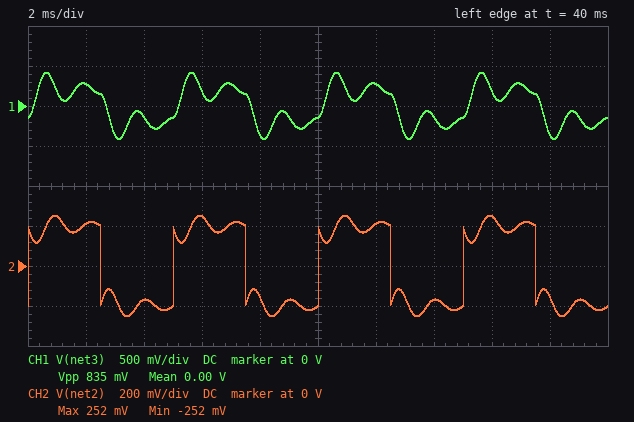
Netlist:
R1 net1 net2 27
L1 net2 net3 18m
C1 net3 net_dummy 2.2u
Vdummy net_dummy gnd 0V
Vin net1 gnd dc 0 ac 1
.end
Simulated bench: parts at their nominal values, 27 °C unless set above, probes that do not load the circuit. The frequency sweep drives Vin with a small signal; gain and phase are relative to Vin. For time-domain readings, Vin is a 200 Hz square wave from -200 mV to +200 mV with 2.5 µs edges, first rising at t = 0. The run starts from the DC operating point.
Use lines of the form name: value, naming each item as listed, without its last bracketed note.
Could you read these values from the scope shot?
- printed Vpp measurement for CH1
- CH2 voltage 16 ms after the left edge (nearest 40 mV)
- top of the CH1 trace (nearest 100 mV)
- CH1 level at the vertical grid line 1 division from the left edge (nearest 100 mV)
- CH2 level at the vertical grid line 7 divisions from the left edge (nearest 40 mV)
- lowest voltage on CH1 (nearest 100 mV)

printed Vpp measurement for CH1: 835 mV
CH2 voltage 16 ms after the left edge: 240 mV
top of the CH1 trace: 400 mV
CH1 level at the vertical grid line 1 division from the left edge: 300 mV
CH2 level at the vertical grid line 7 divisions from the left edge: -160 mV
lowest voltage on CH1: -400 mV
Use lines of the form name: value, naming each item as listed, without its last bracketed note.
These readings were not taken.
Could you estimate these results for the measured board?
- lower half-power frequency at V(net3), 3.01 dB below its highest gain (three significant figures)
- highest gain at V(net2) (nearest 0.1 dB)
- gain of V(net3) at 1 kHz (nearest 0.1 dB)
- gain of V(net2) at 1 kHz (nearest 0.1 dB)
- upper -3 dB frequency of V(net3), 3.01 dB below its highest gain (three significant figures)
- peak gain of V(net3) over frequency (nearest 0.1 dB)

lower half-power frequency at V(net3), 3.01 dB below its highest gain: 650 Hz
highest gain at V(net2): 0 dB
gain of V(net3) at 1 kHz: 3.4 dB
gain of V(net2) at 1 kHz: -1.6 dB
upper -3 dB frequency of V(net3), 3.01 dB below its highest gain: 894 Hz
peak gain of V(net3) over frequency: 10.6 dB
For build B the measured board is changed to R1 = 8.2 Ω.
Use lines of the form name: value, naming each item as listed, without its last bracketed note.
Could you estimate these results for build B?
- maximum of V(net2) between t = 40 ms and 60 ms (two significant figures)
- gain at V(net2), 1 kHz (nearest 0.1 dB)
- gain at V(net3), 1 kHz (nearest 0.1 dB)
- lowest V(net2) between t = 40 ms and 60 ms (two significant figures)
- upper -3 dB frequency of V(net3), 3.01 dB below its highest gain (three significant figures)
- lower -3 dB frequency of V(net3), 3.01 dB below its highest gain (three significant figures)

maximum of V(net2) between t = 40 ms and 60 ms: 220 mV
gain at V(net2), 1 kHz: -0.2 dB
gain at V(net3), 1 kHz: 4.8 dB
lowest V(net2) between t = 40 ms and 60 ms: -220 mV
upper -3 dB frequency of V(net3), 3.01 dB below its highest gain: 834 Hz
lower -3 dB frequency of V(net3), 3.01 dB below its highest gain: 761 Hz
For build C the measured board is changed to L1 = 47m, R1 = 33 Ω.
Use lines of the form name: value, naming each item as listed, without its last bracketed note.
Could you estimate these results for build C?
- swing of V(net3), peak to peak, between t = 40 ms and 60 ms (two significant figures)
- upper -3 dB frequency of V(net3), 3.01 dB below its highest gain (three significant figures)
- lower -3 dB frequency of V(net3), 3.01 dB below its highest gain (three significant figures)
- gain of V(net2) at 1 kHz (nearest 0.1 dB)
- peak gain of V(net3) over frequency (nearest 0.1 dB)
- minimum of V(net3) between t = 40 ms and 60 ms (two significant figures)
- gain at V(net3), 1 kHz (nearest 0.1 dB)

swing of V(net3), peak to peak, between t = 40 ms and 60 ms: 870 mV
upper -3 dB frequency of V(net3), 3.01 dB below its highest gain: 542 Hz
lower -3 dB frequency of V(net3), 3.01 dB below its highest gain: 429 Hz
gain of V(net2) at 1 kHz: -0.1 dB
peak gain of V(net3) over frequency: 13.0 dB
minimum of V(net3) between t = 40 ms and 60 ms: -440 mV
gain at V(net3), 1 kHz: -9.9 dB
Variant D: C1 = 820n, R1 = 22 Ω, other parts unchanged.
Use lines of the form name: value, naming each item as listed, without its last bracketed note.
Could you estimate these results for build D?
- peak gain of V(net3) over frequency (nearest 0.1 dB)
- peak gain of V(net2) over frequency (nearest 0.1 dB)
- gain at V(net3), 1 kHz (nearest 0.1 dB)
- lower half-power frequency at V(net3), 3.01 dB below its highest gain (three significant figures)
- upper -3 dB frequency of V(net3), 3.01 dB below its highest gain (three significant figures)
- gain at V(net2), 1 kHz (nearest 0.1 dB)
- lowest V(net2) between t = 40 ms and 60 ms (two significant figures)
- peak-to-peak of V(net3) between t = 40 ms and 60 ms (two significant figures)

peak gain of V(net3) over frequency: 16.6 dB
peak gain of V(net2) over frequency: 0 dB
gain at V(net3), 1 kHz: 7.3 dB
lower half-power frequency at V(net3), 3.01 dB below its highest gain: 1.20 kHz
upper -3 dB frequency of V(net3), 3.01 dB below its highest gain: 1.40 kHz
gain at V(net2), 1 kHz: -0.3 dB
lowest V(net2) between t = 40 ms and 60 ms: -240 mV
peak-to-peak of V(net3) between t = 40 ms and 60 ms: 1.0 V
